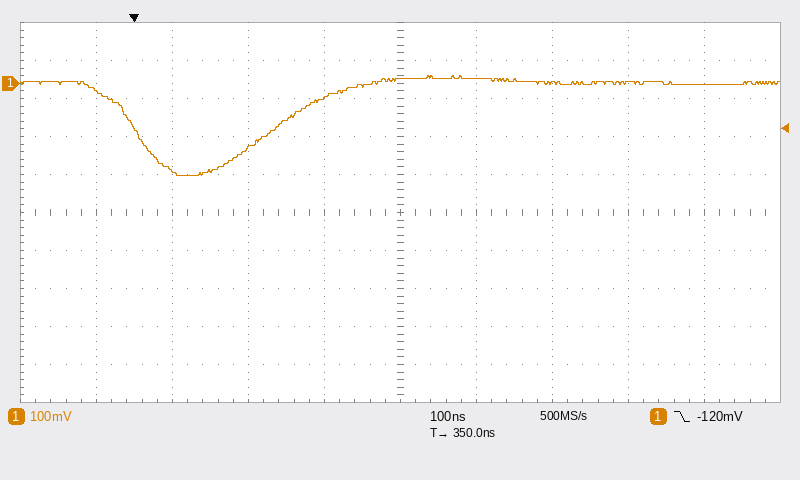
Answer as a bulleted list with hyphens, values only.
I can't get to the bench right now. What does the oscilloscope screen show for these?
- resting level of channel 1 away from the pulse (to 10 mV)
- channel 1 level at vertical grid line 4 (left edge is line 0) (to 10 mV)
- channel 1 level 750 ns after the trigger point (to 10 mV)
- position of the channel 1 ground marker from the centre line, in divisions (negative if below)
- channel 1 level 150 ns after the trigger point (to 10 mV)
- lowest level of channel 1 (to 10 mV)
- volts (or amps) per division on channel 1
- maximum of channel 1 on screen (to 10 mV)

- 0 mV
- -40 mV
- 0 mV
- +3.4 div
- -170 mV
- -240 mV
- 100 mV
- 20 mV
